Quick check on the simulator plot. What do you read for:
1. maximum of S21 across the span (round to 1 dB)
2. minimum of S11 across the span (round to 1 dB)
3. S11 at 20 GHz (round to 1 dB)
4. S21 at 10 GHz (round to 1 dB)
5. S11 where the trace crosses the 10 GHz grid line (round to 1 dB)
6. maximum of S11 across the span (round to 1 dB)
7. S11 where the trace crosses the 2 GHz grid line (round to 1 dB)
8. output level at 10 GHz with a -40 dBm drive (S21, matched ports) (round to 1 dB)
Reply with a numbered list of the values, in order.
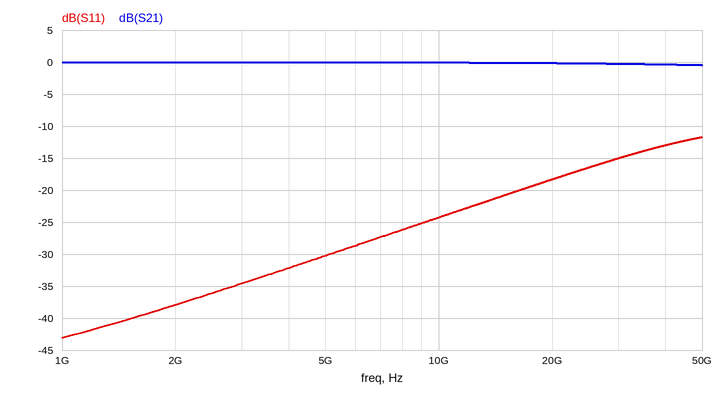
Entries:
1. 0 dB
2. -43 dB
3. -18 dB
4. 0 dB
5. -24 dB
6. -12 dB
7. -38 dB
8. -40 dBm
